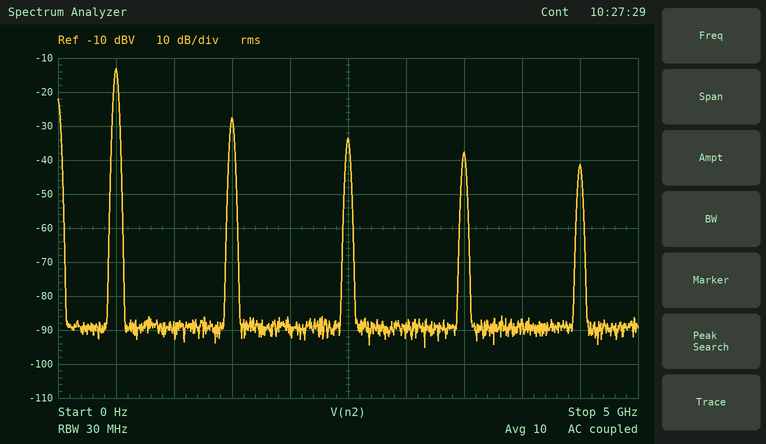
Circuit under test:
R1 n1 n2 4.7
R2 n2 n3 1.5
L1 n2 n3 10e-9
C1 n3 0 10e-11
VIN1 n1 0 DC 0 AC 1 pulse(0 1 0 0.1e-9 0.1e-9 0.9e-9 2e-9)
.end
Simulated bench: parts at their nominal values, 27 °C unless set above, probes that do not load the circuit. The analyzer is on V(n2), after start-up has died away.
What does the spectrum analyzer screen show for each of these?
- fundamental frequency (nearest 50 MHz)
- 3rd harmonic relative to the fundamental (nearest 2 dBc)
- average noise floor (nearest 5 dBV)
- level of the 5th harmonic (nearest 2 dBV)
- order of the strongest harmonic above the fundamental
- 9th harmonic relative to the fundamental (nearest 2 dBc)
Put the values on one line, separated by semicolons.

500 MHz; -14 dBc; -90 dBV; -34 dBV; 3; -28 dBc
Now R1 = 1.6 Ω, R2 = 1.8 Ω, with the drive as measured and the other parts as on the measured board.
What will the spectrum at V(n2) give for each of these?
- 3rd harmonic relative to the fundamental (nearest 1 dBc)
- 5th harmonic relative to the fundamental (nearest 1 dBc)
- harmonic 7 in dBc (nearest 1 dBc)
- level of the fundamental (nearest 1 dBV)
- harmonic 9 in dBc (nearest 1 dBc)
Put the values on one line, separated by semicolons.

-12 dBc; -18 dBc; -22 dBc; -9 dBV; -25 dBc
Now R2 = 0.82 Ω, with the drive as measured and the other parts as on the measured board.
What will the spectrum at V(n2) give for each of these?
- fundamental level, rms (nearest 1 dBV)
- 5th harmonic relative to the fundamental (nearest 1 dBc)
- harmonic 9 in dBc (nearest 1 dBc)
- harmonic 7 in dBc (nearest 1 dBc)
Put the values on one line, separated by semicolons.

-13 dBV; -24 dBc; -32 dBc; -28 dBc
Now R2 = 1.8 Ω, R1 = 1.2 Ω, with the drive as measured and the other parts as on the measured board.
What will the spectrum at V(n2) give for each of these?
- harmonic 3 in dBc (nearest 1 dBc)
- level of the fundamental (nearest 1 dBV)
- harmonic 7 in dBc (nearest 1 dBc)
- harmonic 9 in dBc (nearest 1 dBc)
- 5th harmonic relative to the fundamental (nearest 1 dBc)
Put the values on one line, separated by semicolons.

-12 dBc; -9 dBV; -21 dBc; -25 dBc; -17 dBc
